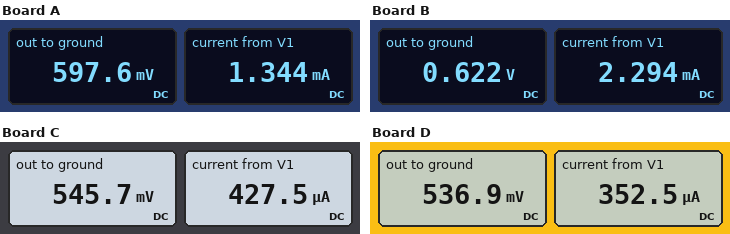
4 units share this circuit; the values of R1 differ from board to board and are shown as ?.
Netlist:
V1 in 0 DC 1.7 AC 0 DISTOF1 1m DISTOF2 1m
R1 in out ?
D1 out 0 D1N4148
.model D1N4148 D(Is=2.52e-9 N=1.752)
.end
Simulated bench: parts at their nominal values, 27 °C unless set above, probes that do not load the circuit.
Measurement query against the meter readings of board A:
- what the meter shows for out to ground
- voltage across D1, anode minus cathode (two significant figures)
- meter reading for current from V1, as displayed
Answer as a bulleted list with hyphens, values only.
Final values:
- 597.6 mV
- 600 mV
- 1.344 mA
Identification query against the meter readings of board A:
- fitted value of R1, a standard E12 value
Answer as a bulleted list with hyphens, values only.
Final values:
- 820 Ω
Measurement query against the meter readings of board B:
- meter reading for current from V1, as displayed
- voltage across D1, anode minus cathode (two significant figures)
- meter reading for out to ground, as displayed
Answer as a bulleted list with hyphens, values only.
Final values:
- 2.294 mA
- 620 mV
- 0.622 V
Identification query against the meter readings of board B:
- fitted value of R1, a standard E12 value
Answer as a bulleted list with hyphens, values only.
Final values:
- 470 Ω
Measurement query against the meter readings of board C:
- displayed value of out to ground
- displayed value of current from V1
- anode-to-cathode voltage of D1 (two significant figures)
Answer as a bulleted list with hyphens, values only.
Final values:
- 545.7 mV
- 427.5 µA
- 550 mV
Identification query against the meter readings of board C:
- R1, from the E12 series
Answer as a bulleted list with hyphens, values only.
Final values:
- 2.7 kΩ
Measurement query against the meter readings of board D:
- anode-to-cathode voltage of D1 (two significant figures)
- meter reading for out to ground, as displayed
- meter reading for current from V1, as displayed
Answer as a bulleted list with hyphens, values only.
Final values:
- 540 mV
- 536.9 mV
- 352.5 µA
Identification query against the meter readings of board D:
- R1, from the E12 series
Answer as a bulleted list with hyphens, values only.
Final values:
- 3.3 kΩ
